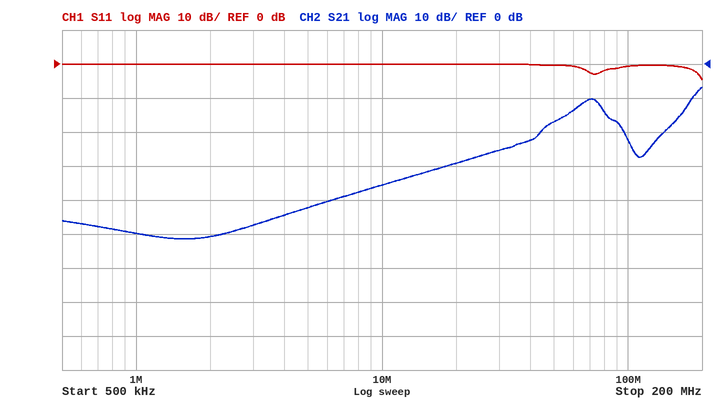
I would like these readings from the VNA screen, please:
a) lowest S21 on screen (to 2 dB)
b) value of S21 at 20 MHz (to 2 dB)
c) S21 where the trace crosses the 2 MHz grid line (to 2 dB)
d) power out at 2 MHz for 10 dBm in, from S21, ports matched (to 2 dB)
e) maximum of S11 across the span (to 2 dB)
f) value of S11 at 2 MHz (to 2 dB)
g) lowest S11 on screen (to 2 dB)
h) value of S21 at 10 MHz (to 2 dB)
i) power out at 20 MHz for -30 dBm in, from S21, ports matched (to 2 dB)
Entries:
-52 dB
-30 dB
-50 dB
-40 dBm
0 dB
0 dB
-4 dB
-36 dB
-60 dBm
